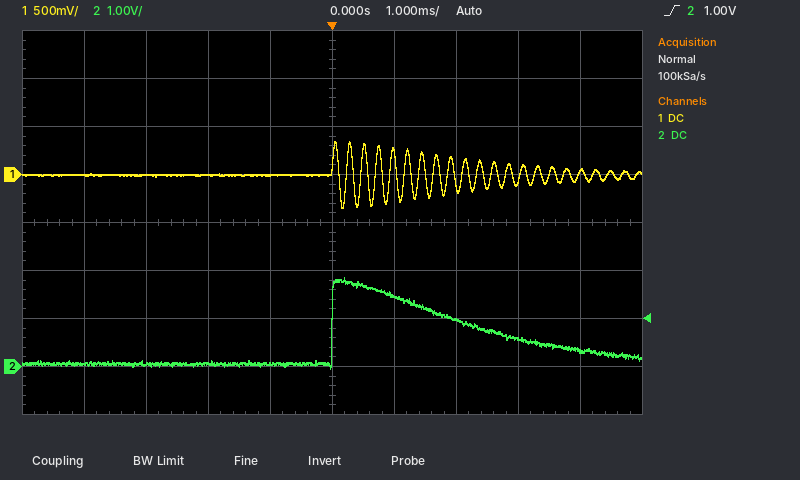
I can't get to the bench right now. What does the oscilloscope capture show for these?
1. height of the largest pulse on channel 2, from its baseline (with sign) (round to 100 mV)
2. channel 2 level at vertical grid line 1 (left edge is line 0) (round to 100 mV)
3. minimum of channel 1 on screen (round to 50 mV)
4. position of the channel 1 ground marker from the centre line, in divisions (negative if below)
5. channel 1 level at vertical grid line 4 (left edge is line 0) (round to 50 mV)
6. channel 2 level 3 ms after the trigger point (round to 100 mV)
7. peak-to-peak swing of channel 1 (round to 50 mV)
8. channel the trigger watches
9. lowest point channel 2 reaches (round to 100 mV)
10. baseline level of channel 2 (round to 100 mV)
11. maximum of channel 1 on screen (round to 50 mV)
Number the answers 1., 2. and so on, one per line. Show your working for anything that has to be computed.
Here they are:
1. +1.8 V
2. 100 mV
3. -350 mV
4. +1.0 div
5. 0 mV
6. 600 mV
7. 350 mV − (-350 mV) = 700 mV
8. channel 2
9. 0.0 V
10. 100 mV
11. 350 mV
